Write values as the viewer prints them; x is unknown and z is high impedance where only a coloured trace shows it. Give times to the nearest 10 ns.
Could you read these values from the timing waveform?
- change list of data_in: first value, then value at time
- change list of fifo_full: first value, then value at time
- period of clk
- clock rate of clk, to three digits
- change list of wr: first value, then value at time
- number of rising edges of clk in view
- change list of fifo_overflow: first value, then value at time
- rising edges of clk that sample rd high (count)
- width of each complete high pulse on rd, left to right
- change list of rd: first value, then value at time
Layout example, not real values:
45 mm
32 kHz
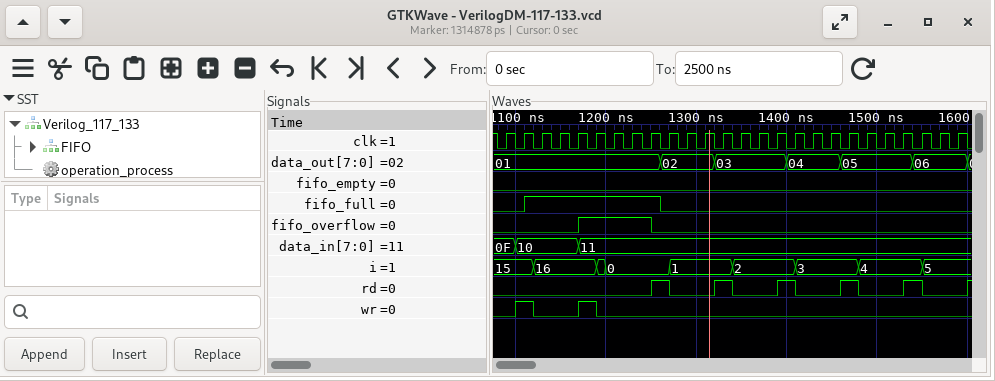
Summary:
0F, 10 at 1100 ns, 11 at 1170 ns
0, 1 at 1110 ns, 0 at 1260 ns
20 ns
50.0 MHz
0, 1 at 1100 ns, 0 at 1120 ns, 1 at 1170 ns, 0 at 1190 ns
26
0, 1 at 1170 ns, 0 at 1250 ns
5
20 ns, 20 ns, 20 ns, 20 ns, 20 ns
0, 1 at 1250 ns, 0 at 1270 ns, 1 at 1320 ns, 0 at 1340 ns, 1 at 1390 ns, 0 at 1410 ns, 1 at 1460 ns, 0 at 1480 ns, 1 at 1530 ns, 0 at 1550 ns, 1 at 1600 ns
